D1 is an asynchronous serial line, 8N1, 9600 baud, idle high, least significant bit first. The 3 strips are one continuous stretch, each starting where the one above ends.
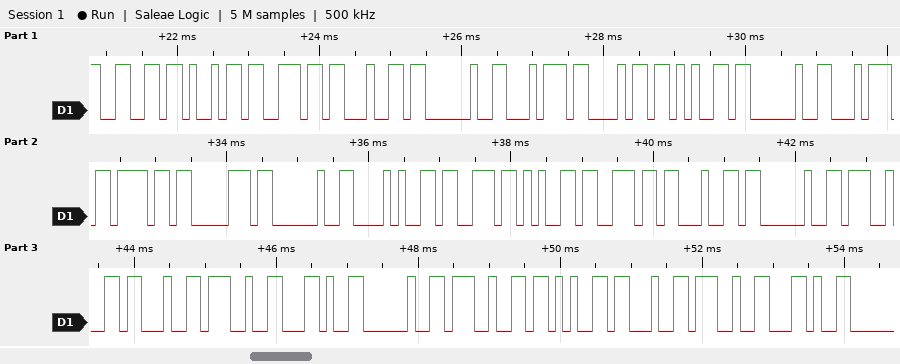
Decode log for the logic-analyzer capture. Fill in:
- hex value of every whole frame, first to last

66 69 6E 64 20 74 68 65 20 74 6F 70 20 28 73 65 6E 64 20 27 23 27 2C 20 27 2B 23 27 2C
